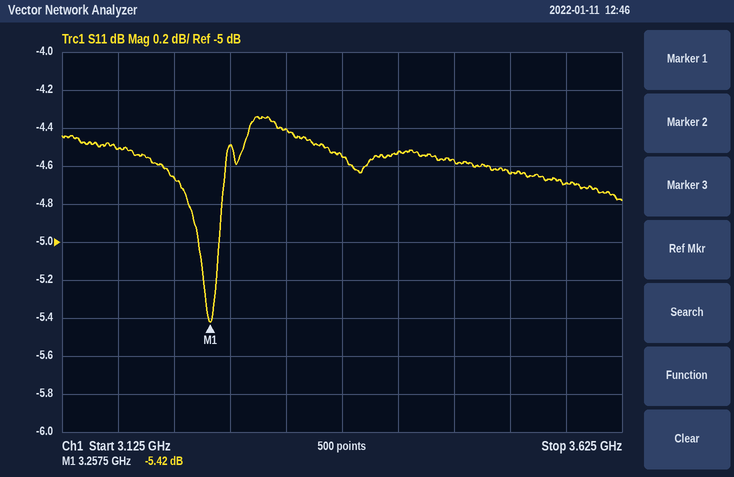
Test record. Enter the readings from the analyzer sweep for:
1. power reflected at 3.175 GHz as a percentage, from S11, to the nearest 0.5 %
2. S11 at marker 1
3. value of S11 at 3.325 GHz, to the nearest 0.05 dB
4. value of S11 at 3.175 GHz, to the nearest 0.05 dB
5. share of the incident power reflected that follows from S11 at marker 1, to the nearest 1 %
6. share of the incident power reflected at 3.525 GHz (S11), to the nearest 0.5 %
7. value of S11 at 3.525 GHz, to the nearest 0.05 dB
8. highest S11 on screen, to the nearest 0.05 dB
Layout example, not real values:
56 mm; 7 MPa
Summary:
35.5 %; -5.42 dB; -4.40 dB; -4.50 dB; 29 %; 34.5 %; -4.65 dB; -4.35 dB
